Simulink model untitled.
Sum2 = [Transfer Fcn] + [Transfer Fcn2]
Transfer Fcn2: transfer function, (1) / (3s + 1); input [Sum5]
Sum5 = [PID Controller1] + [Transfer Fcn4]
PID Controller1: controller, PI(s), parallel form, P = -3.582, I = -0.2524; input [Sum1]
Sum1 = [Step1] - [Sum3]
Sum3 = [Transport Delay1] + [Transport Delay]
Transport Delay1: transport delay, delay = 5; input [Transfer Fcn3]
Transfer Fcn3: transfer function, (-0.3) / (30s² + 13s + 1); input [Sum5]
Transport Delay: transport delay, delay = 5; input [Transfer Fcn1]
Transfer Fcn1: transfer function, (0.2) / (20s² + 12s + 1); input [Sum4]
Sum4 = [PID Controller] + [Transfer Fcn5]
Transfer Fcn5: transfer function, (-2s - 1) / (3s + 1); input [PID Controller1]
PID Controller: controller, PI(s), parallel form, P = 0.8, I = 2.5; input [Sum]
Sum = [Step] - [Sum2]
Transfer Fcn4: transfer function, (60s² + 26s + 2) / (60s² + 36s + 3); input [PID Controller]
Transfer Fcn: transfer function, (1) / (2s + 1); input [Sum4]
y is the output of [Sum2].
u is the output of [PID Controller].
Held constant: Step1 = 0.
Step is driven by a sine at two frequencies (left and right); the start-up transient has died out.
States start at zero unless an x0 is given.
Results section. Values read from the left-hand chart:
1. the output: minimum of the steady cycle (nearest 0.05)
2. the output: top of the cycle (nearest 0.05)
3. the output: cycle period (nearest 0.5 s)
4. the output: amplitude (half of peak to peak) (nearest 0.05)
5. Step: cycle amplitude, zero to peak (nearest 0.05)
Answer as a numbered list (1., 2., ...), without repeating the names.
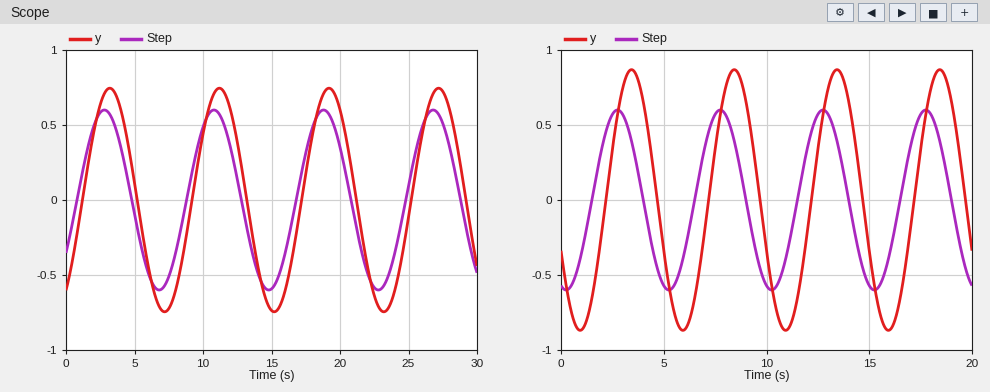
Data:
1. -0.75
2. 0.75
3. 8.0 s
4. 0.75
5. 0.60
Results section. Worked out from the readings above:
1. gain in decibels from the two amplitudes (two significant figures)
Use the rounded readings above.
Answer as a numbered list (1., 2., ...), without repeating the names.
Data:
1. 1.9 dB
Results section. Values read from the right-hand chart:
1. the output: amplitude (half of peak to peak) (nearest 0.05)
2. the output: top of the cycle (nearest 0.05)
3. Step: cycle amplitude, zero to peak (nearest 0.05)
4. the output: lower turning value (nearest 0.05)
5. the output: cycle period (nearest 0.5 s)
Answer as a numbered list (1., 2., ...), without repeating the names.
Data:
1. 0.85
2. 0.85
3. 0.60
4. -0.85
5. 5.0 s
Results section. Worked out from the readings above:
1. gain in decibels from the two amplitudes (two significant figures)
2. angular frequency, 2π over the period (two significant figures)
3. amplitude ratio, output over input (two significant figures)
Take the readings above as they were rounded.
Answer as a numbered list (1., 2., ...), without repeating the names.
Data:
1. 3.0 dB
2. 1.3 rad/s
3. 1.4
